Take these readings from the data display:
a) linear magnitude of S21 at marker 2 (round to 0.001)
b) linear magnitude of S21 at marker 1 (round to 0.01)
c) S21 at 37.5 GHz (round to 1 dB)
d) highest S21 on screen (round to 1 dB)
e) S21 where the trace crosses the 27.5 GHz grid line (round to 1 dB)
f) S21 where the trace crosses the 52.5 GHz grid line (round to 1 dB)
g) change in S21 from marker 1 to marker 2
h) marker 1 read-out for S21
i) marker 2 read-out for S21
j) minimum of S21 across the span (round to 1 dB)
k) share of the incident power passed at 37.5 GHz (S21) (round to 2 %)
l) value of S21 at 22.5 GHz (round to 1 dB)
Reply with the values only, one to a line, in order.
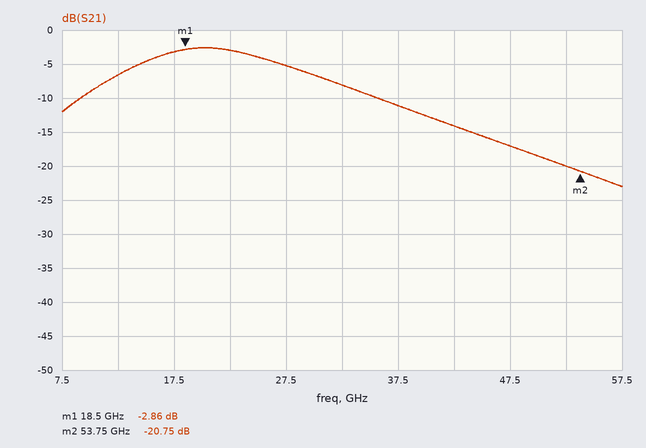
0.092
0.72
-11 dB
-3 dB
-5 dB
-20 dB
-17.89 dB
-2.86 dB
-20.75 dB
-23 dB
8 %
-3 dB
